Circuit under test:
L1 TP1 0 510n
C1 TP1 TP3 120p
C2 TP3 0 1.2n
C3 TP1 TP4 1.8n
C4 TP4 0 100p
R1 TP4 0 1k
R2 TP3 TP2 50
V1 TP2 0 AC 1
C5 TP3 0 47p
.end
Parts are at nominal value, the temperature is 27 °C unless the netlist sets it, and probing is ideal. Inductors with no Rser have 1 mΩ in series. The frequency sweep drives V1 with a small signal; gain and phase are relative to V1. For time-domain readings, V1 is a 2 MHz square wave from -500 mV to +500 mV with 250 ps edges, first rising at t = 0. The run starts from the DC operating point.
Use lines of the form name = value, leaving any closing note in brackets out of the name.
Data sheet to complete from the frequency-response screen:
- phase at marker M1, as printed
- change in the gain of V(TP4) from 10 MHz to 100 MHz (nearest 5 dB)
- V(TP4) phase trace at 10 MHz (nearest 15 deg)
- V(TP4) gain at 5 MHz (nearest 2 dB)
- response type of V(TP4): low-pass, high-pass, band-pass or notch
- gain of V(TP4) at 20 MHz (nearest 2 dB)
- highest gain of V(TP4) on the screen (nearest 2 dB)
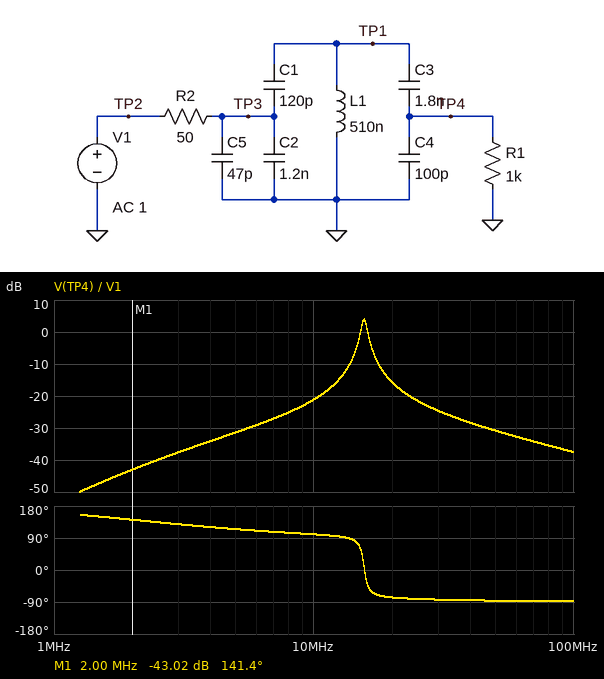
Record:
phase at marker M1, as printed = 141.4 deg
change in the gain of V(TP4) from 10 MHz to 100 MHz = -15 dB
V(TP4) phase trace at 10 MHz = 105 deg
V(TP4) gain at 5 MHz = -32 dB
response type of V(TP4): low-pass, high-pass, band-pass or notch = band-pass
gain of V(TP4) at 20 MHz = -16 dB
highest gain of V(TP4) on the screen = 4 dB
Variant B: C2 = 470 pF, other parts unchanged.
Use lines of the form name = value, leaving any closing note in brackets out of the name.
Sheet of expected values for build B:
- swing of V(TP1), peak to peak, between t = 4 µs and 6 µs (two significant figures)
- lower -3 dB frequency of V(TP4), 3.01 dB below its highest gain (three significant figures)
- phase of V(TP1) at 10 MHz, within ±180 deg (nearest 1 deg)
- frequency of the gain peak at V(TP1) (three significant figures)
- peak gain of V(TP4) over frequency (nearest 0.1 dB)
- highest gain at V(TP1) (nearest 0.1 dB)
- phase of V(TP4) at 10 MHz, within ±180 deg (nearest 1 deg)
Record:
swing of V(TP1), peak to peak, between t = 4 µs and 6 µs = 260 mV
lower -3 dB frequency of V(TP4), 3.01 dB below its highest gain = 15.4 MHz
phase of V(TP1) at 10 MHz, within ±180 deg = 112 deg
frequency of the gain peak at V(TP1) = 16.0 MHz
peak gain of V(TP4) over frequency = 6.9 dB
highest gain at V(TP1) = 7.3 dB
phase of V(TP4) at 10 MHz, within ±180 deg = 113 deg
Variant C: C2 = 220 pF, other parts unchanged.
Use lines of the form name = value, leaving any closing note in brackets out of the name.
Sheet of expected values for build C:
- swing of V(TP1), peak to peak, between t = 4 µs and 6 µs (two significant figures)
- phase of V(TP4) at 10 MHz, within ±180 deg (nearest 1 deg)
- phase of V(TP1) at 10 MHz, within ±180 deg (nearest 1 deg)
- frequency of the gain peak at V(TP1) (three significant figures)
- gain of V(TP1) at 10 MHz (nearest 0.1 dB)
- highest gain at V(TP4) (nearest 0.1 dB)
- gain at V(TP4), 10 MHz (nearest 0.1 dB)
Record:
swing of V(TP1), peak to peak, between t = 4 µs and 6 µs = 430 mV
phase of V(TP4) at 10 MHz, within ±180 deg = 124 deg
phase of V(TP1) at 10 MHz, within ±180 deg = 123 deg
frequency of the gain peak at V(TP1) = 16.4 MHz
gain of V(TP1) at 10 MHz = -12.1 dB
highest gain at V(TP4) = 6.7 dB
gain at V(TP4), 10 MHz = -12.5 dB
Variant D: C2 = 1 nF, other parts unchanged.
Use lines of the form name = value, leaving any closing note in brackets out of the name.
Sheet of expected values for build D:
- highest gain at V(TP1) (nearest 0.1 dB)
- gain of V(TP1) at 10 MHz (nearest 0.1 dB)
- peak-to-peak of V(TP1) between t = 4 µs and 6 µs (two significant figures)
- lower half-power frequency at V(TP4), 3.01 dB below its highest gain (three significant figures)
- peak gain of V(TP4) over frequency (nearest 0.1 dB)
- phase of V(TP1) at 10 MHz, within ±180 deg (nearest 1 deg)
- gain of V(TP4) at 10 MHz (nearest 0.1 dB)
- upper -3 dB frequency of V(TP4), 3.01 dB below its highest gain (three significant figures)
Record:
highest gain at V(TP1) = 5.3 dB
gain of V(TP1) at 10 MHz = -19.4 dB
peak-to-peak of V(TP1) between t = 4 µs and 6 µs = 140 mV
lower half-power frequency at V(TP4), 3.01 dB below its highest gain = 15.2 MHz
peak gain of V(TP4) over frequency = 4.8 dB
phase of V(TP1) at 10 MHz, within ±180 deg = 102 deg
gain of V(TP4) at 10 MHz = -19.8 dB
upper -3 dB frequency of V(TP4), 3.01 dB below its highest gain = 16.1 MHz
